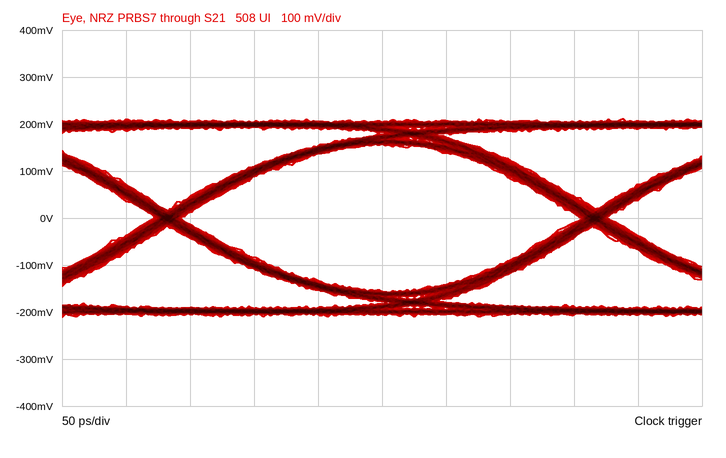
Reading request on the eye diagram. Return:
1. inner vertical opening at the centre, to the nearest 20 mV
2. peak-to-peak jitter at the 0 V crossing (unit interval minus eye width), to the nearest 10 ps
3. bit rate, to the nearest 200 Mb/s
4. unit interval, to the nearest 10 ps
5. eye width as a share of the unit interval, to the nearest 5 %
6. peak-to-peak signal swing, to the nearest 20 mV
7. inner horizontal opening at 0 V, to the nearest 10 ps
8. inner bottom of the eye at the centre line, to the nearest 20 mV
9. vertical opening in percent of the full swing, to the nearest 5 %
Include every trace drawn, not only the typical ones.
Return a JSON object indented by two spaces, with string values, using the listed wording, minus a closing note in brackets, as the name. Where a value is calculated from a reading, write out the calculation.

{
  "inner vertical opening at the centre, to the nearest 20 mV": "320 mV",
  "peak-to-peak jitter at the 0 V crossing (unit interval minus eye width), to the nearest 10 ps": "20 ps",
  "bit rate, to the nearest 200 Mb/s": "3.0 Gb/s",
  "unit interval, to the nearest 10 ps": "330 ps",
  "eye width as a share of the unit interval, to the nearest 5 %": "310 ps / 330 ps ≈ 93.9 %, so 95 % to the nearest 5 %",
  "peak-to-peak signal swing, to the nearest 20 mV": "420 mV",
  "inner horizontal opening at 0 V, to the nearest 10 ps": "310 ps",
  "inner bottom of the eye at the centre line, to the nearest 20 mV": "-160 mV",
  "vertical opening in percent of the full swing, to the nearest 5 %": "320 mV / 420 mV ≈ 76.2 %, so 75 % to the nearest 5 %"
}
